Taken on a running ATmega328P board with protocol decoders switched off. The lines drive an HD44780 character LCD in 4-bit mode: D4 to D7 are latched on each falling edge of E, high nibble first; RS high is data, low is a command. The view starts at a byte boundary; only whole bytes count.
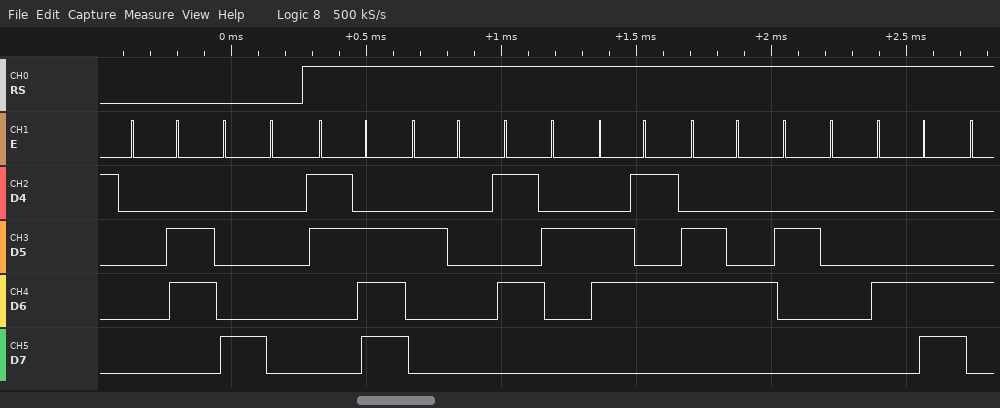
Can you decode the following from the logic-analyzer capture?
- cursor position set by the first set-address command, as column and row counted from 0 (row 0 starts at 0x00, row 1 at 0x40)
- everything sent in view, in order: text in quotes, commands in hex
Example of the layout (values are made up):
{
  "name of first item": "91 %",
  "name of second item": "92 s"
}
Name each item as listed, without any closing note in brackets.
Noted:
{
  "cursor position set by the first set-address command, as column and row counted from 0": "column 0, row 0",
  "everything sent in view, in order: text in quotes, commands in hex": "0x06 0x80 \"> Red L\""
}
